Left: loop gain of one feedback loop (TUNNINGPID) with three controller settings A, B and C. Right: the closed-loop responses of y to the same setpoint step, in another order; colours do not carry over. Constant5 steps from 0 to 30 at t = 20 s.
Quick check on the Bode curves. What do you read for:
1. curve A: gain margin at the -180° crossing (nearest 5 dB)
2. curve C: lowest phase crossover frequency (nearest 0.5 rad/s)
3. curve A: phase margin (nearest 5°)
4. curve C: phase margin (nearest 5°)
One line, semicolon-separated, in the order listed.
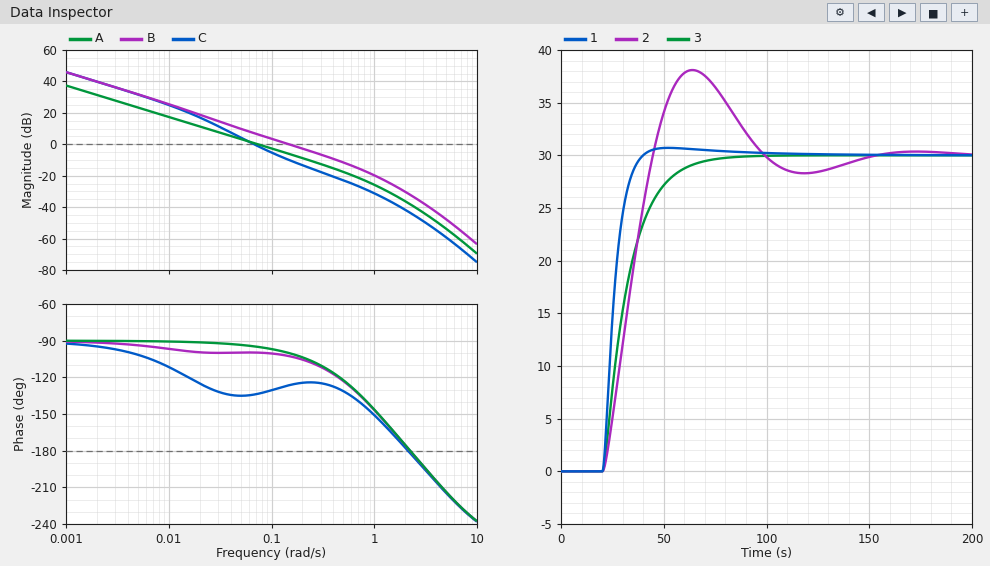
40 dB; 2.0 rad/s; 85°; 45°
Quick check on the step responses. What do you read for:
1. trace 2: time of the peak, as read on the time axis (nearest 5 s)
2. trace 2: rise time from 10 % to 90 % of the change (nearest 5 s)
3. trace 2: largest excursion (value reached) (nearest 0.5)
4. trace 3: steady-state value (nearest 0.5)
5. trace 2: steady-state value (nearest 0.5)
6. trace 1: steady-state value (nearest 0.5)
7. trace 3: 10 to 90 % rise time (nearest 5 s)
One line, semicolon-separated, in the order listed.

65 s; 20 s; 38.0; 30.0; 30.0; 30.0; 25 s
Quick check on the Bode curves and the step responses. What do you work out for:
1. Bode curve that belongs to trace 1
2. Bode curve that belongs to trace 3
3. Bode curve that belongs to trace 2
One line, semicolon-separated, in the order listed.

B; A; C
